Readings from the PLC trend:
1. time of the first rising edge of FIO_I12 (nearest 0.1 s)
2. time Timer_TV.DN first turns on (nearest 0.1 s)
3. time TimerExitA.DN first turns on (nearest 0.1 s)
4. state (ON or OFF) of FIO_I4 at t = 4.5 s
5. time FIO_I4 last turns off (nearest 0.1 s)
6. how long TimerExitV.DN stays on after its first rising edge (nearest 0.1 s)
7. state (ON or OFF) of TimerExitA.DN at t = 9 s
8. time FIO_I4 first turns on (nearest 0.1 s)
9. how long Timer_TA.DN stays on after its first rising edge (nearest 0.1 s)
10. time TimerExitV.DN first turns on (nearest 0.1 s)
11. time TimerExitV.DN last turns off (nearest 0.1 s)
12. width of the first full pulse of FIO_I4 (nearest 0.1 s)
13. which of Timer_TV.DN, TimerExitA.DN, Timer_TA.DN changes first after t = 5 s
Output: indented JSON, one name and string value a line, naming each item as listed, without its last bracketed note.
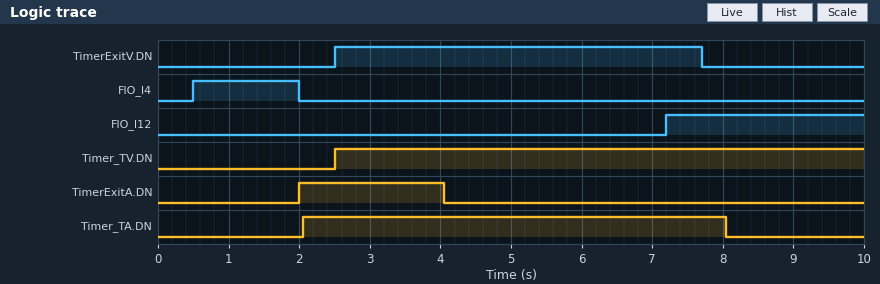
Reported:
{
  "time of the first rising edge of FIO_I12": "7.2 s",
  "time Timer_TV.DN first turns on": "2.5 s",
  "time TimerExitA.DN first turns on": "2.0 s",
  "state (ON or OFF) of FIO_I4 at t = 4.5 s": "OFF",
  "time FIO_I4 last turns off": "2.0 s",
  "how long TimerExitV.DN stays on after its first rising edge": "5.2 s",
  "state (ON or OFF) of TimerExitA.DN at t = 9 s": "OFF",
  "time FIO_I4 first turns on": "0.5 s",
  "how long Timer_TA.DN stays on after its first rising edge": "6.0 s",
  "time TimerExitV.DN first turns on": "2.5 s",
  "time TimerExitV.DN last turns off": "7.7 s",
  "width of the first full pulse of FIO_I4": "1.5 s",
  "which of Timer_TV.DN, TimerExitA.DN, Timer_TA.DN changes first after t = 5 s": "Timer_TA.DN"
}
